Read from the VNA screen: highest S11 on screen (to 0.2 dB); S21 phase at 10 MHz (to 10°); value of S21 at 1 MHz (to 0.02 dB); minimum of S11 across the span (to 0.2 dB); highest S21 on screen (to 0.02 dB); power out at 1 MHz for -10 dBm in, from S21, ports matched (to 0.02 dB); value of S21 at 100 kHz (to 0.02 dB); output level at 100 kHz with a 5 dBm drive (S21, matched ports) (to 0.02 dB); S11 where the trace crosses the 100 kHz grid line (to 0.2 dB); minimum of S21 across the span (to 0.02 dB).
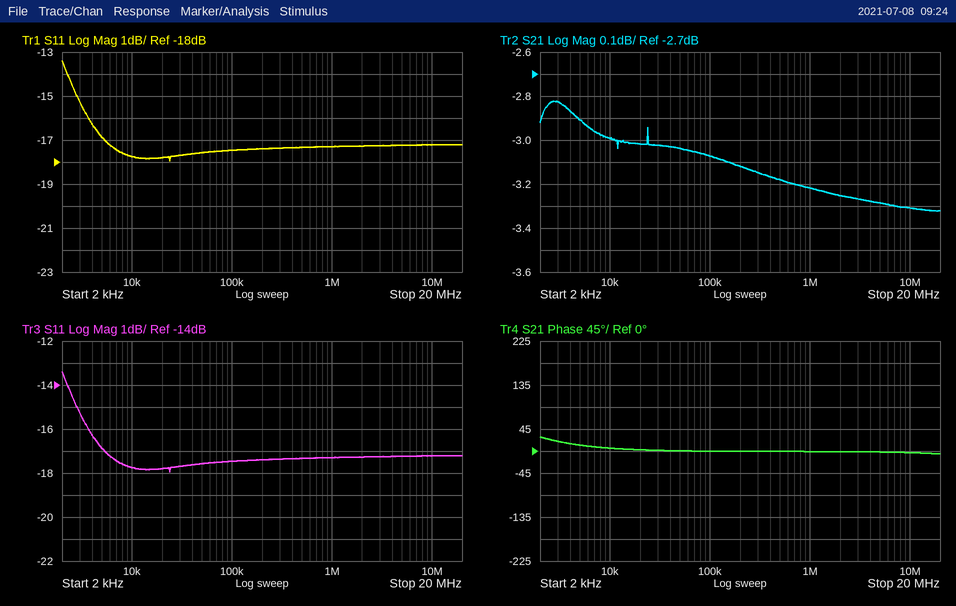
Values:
-13.4 dB
0°
-3.22 dB
-18.0 dB
-2.82 dB
-13.22 dBm
-3.08 dB
1.92 dBm
-17.4 dB
-3.32 dB
